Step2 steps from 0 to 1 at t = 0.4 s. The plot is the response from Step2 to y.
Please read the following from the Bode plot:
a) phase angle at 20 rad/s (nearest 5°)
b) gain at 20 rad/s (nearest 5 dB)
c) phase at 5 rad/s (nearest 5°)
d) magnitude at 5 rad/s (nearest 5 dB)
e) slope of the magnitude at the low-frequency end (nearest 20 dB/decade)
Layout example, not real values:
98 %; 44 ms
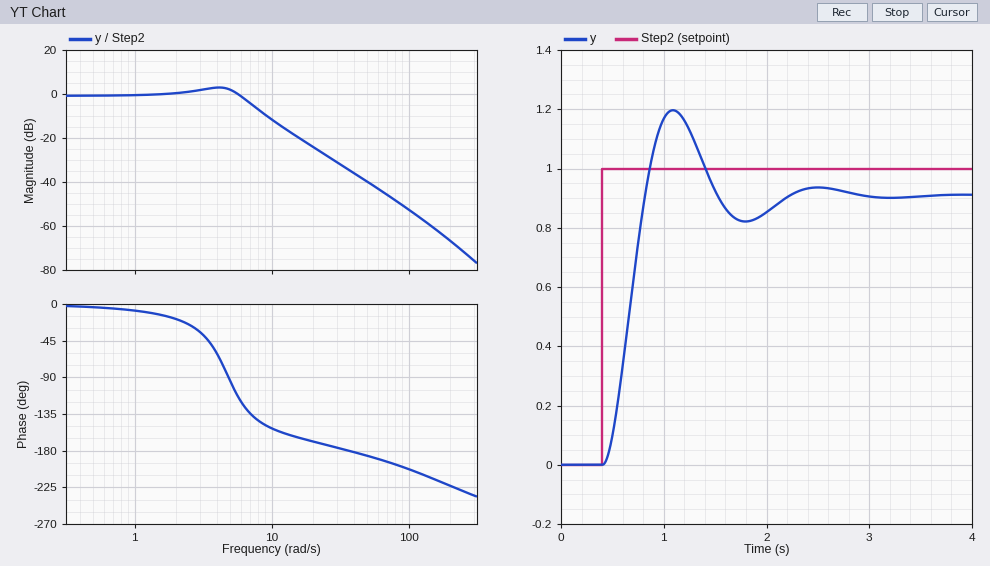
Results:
-170°; -25 dB; -95°; 0 dB; 0 dB/decade
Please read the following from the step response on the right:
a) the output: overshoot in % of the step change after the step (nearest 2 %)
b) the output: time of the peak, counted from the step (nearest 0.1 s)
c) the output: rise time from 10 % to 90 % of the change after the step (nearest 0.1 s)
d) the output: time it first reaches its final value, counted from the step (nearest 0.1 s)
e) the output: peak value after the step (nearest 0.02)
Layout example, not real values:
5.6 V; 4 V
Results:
32 %; 0.7 s; 0.3 s; 0.4 s; 1.20
